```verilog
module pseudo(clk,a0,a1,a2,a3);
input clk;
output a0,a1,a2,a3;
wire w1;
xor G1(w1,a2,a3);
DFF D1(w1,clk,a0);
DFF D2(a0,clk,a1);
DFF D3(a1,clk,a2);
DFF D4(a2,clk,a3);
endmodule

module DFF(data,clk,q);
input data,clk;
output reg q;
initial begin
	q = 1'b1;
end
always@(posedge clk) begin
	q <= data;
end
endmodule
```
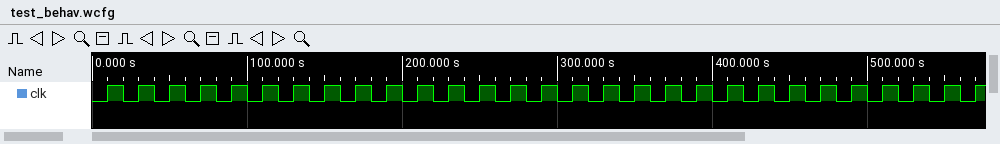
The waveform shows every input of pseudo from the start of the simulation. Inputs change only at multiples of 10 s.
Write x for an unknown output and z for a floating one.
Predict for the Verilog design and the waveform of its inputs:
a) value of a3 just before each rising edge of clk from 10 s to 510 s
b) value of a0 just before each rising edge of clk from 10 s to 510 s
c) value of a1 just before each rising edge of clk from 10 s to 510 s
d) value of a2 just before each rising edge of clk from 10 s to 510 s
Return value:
1 1 1 1 0 0 0 1 0 0 1 1 0 1 0 1 1 1 1 0 0 0 1 0 0 1
1 0 0 0 1 0 0 1 1 0 1 0 1 1 1 1 0 0 0 1 0 0 1 1 0 1
1 1 0 0 0 1 0 0 1 1 0 1 0 1 1 1 1 0 0 0 1 0 0 1 1 0
1 1 1 0 0 0 1 0 0 1 1 0 1 0 1 1 1 1 0 0 0 1 0 0 1 1
